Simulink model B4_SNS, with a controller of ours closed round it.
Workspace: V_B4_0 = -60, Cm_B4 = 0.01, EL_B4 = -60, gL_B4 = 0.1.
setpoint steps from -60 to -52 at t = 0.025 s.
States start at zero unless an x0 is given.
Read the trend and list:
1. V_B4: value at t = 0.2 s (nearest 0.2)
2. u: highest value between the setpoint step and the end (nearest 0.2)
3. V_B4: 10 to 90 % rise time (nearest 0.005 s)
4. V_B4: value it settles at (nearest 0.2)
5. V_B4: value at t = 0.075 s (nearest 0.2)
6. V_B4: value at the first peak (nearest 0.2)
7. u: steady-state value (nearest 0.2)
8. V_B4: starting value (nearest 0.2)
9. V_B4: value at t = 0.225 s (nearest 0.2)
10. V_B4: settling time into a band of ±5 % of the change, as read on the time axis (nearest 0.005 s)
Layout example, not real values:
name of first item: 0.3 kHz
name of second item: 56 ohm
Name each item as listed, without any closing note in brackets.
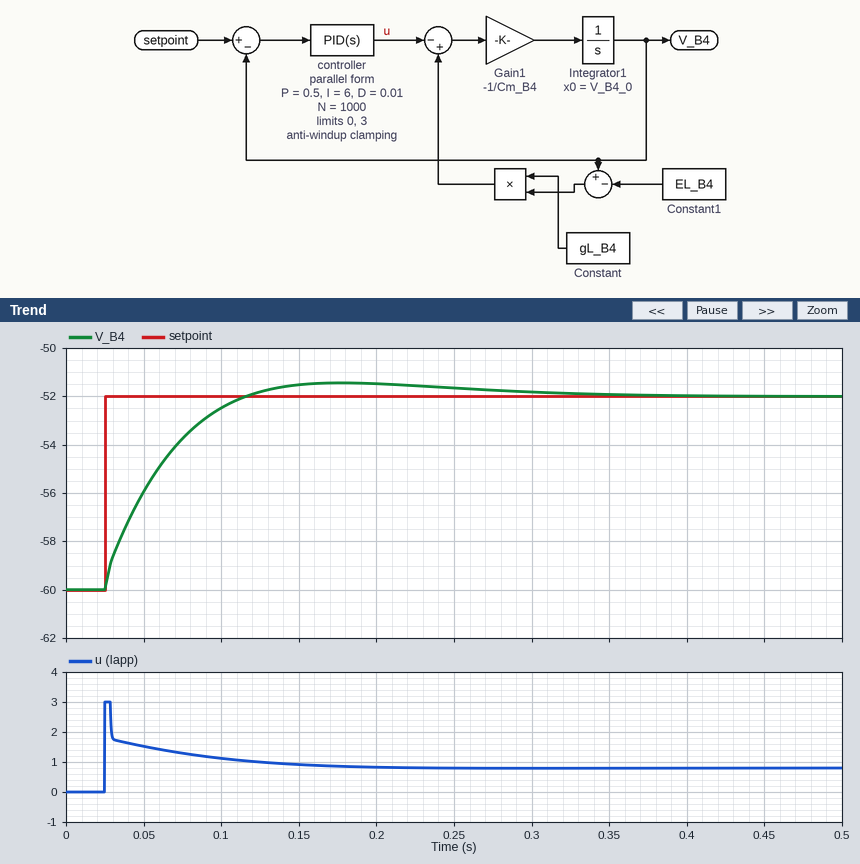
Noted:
V_B4: value at t = 0.2 s: -51.4
u: highest value between the setpoint step and the end: 3.0
V_B4: 10 to 90 % rise time: 0.065 s
V_B4: value it settles at: -52.0
V_B4: value at t = 0.075 s: -53.8
V_B4: value at the first peak: -51.4
u: steady-state value: 0.8
V_B4: starting value: -60.0
V_B4: value at t = 0.225 s: -51.6
V_B4: settling time into a band of ±5 % of the change, as read on the time axis: 0.235 s
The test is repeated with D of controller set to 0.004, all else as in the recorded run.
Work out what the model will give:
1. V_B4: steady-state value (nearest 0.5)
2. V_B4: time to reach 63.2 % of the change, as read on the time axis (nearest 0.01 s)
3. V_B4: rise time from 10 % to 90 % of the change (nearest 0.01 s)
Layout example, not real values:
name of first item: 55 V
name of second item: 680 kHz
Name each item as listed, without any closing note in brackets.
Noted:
V_B4: steady-state value: -52.0
V_B4: time to reach 63.2 % of the change, as read on the time axis: 0.05 s
V_B4: rise time from 10 % to 90 % of the change: 0.05 s
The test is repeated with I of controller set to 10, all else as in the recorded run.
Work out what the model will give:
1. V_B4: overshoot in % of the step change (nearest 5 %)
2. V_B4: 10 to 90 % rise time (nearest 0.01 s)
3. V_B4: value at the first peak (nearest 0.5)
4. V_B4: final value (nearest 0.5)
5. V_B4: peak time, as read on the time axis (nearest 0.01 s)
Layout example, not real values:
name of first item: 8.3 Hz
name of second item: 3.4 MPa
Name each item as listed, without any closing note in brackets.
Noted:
V_B4: overshoot in % of the step change: 15 %
V_B4: 10 to 90 % rise time: 0.05 s
V_B4: value at the first peak: -51.0
V_B4: final value: -52.0
V_B4: peak time, as read on the time axis: 0.14 s
